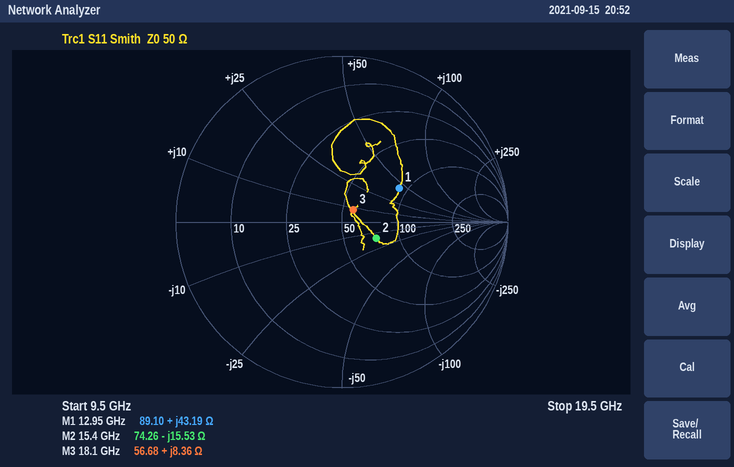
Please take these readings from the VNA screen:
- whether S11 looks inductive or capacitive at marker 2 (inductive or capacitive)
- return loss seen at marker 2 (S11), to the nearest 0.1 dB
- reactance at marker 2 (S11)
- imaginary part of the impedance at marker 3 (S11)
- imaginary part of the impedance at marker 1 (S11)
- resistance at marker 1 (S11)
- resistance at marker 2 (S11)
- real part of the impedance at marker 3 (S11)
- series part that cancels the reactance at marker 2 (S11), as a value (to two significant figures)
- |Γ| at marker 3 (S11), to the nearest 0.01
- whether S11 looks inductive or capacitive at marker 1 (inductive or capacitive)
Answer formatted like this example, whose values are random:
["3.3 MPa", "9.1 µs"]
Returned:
["capacitive", "12.8 dB", "-15.53 Ω", "+8.36 Ω", "+43.19 Ω", "89.10 Ω", "74.26 Ω", "56.68 Ω", "160 pH", "0.10", "inductive"]
